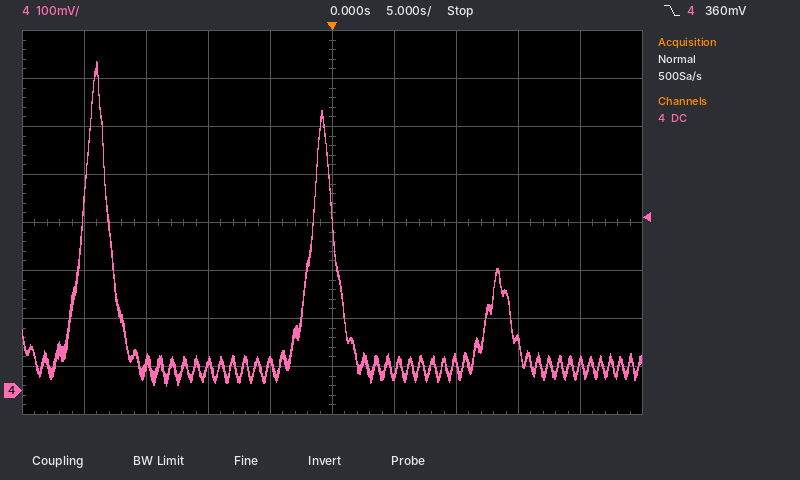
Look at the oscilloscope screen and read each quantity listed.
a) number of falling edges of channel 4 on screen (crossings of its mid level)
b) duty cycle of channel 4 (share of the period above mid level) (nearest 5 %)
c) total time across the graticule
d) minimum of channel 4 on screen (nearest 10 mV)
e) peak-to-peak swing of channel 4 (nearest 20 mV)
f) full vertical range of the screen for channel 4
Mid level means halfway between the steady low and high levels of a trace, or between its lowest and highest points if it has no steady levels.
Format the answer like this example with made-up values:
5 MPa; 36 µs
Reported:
2; 10 %; 50 s; 10 mV; 680 mV; 800 mV
